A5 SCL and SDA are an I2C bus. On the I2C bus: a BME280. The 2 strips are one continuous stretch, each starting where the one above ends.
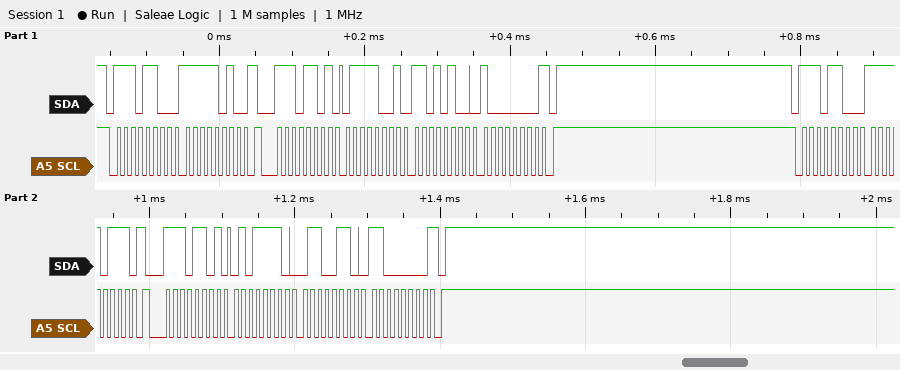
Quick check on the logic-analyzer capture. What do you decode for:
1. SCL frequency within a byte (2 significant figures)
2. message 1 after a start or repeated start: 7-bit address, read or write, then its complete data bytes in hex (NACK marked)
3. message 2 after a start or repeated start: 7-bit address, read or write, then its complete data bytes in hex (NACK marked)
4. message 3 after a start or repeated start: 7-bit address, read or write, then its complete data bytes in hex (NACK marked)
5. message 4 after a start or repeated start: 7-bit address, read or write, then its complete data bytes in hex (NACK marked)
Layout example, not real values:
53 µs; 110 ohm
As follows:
100 kHz; 0x76 write: FA; 0x76 read: 79 D4 80 NACK; 0x76 write: F7; 0x76 read: 5E 66 C0 NACK
